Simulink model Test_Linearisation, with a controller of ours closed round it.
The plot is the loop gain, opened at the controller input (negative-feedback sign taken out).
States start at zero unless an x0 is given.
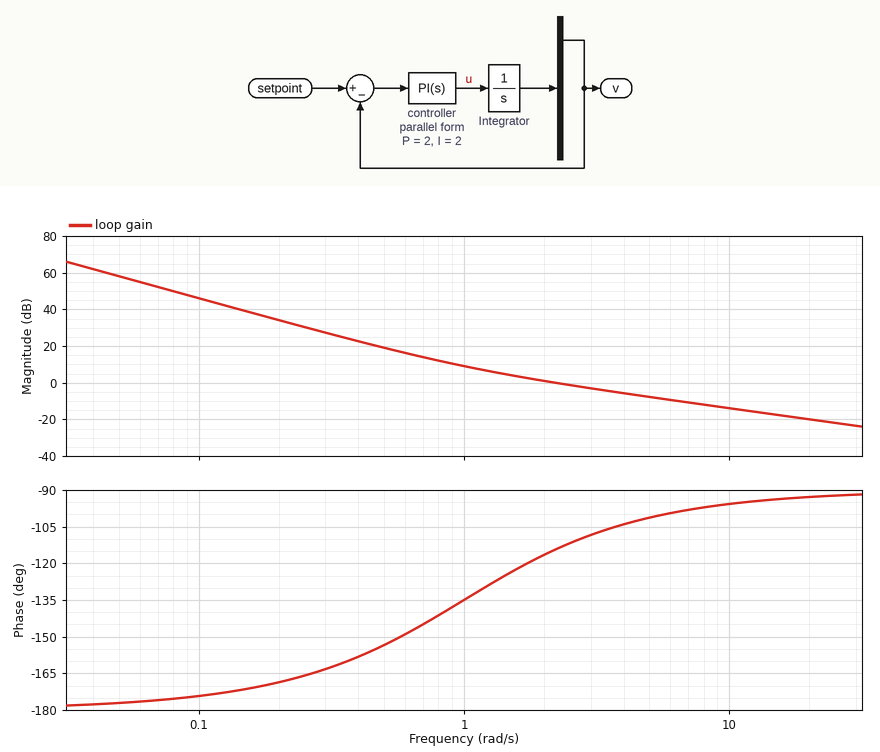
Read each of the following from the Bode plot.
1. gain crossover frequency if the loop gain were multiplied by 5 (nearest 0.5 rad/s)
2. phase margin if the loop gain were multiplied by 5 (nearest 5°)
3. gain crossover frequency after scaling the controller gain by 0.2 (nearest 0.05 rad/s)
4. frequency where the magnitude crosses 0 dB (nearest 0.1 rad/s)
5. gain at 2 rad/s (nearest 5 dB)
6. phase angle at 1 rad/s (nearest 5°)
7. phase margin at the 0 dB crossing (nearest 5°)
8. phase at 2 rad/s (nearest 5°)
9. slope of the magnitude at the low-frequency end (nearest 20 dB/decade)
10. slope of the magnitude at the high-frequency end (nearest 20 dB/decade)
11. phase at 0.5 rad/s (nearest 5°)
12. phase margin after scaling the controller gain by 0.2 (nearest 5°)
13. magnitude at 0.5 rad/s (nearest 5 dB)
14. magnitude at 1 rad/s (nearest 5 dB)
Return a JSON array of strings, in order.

["10.0 rad/s", "85°", "0.70 rad/s", "2.2 rad/s", "0 dB", "-135°", "65°", "-115°", "-40 dB/decade", "-20 dB/decade", "-155°", "35°", "20 dB", "10 dB"]
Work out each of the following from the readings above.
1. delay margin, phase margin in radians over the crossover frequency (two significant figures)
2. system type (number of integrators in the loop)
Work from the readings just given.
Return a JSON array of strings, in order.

["0.52 s", "2"]
